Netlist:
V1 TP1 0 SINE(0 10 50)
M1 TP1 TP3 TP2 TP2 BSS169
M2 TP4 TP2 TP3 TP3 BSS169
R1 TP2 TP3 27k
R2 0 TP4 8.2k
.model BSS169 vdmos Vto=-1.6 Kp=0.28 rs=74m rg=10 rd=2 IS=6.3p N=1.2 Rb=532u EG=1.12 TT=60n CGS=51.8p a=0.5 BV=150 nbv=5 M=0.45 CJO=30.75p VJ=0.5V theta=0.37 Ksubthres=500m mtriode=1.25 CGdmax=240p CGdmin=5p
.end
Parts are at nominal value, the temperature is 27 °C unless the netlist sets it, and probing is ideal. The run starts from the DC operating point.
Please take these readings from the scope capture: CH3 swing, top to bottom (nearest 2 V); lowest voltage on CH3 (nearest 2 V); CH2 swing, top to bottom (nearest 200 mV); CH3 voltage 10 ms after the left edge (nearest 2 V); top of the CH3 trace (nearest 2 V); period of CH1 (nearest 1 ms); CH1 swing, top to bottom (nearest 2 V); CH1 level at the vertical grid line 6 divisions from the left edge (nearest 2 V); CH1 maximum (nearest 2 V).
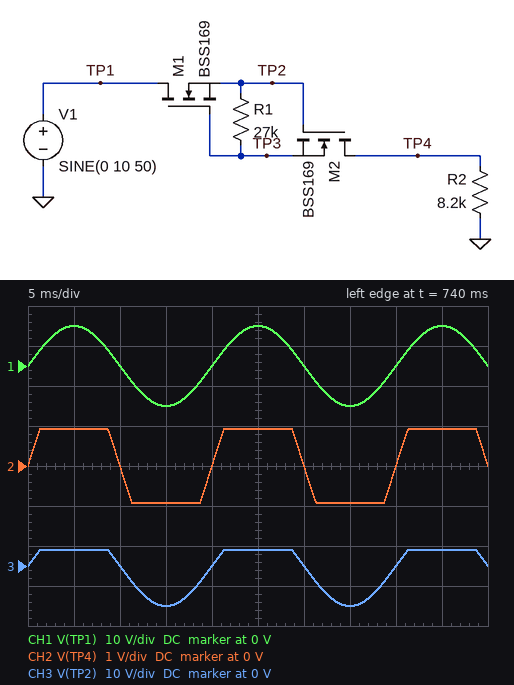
14 V
-10 V
1.8 V
0 V
4 V
20 ms
20 V
0 V
10 V
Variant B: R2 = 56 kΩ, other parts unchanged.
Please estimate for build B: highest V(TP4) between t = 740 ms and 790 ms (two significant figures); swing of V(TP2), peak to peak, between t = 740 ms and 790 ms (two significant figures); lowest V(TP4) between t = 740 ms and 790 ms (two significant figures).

6.3 V
19 V
-6.3 V
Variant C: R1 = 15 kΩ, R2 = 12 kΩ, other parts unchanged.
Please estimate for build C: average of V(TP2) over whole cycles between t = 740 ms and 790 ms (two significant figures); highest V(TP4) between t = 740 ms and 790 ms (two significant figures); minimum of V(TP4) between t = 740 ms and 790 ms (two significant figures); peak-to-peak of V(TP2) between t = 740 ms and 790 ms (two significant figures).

-1.0 V
2.3 V
-2.3 V
15 V
